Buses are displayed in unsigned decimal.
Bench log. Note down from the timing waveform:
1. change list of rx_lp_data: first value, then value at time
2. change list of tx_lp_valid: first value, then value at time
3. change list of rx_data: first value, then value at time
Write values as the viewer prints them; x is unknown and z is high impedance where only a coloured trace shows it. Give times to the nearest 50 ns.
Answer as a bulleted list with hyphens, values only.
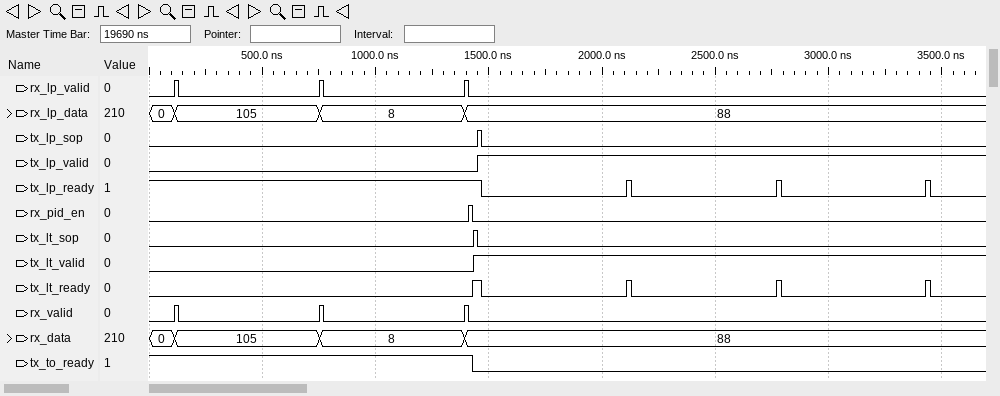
- 0, 105 at 100 ns, 8 at 750 ns, 88 at 1400 ns
- 0, 1 at 1450 ns
- 0, 105 at 100 ns, 8 at 750 ns, 88 at 1400 ns
